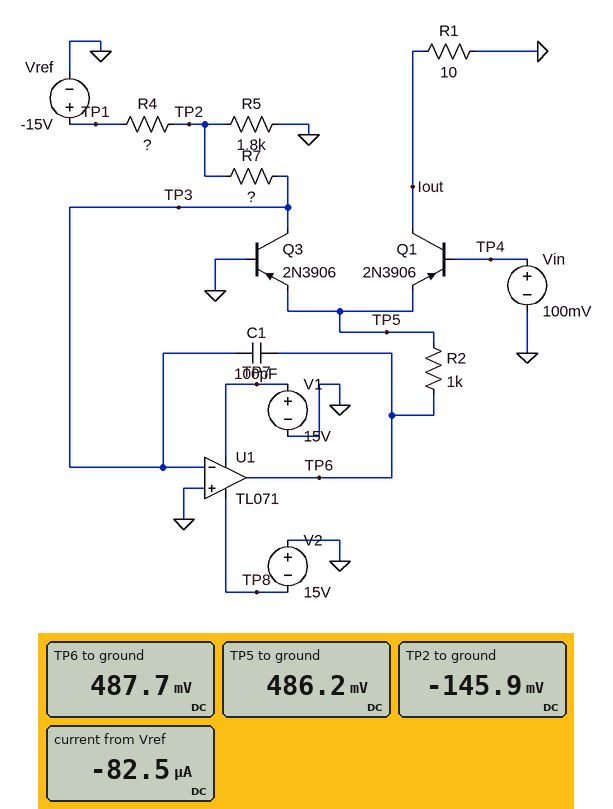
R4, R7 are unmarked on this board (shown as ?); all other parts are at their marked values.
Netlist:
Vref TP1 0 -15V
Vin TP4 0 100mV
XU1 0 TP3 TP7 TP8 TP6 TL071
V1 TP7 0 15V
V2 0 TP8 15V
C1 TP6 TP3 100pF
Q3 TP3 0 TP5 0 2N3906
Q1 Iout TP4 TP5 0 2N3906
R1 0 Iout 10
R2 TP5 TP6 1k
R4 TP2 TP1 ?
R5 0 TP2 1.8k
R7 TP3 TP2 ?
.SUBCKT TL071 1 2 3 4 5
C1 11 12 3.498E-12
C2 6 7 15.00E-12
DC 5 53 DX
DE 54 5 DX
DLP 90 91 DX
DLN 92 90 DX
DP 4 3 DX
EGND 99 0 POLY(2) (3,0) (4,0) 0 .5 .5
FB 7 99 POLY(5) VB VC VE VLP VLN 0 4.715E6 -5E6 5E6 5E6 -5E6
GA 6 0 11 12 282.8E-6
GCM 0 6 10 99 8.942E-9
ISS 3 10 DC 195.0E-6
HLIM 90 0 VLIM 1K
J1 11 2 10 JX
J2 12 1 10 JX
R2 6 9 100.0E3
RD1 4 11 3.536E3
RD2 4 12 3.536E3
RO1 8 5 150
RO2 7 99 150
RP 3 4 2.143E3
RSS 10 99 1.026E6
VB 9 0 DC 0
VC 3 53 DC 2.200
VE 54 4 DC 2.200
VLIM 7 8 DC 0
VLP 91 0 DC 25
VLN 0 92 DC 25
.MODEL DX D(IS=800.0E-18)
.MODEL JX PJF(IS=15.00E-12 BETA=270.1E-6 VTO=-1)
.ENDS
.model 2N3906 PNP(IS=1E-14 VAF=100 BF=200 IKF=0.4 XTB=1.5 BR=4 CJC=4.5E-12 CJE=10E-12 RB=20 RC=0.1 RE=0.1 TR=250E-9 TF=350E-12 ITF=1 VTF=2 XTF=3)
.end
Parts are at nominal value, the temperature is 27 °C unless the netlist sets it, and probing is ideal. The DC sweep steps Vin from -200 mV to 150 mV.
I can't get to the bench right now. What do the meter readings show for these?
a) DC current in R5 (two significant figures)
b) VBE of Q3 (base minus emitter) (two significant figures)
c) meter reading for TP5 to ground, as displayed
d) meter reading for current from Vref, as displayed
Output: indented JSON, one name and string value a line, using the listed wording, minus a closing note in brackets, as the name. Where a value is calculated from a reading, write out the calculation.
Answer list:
{
  "DC current in R5": "(0 V - (-145.9 mV)) / 1.8 kΩ = 81 µA",
  "VBE of Q3 (base minus emitter)": "0 V - 486.2 mV = -490 mV",
  "meter reading for TP5 to ground, as displayed": "486.2 mV",
  "meter reading for current from Vref, as displayed": "-82.5 µA"
}
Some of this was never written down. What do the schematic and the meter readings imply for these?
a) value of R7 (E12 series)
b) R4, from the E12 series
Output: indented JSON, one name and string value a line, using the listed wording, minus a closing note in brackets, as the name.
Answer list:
{
  "value of R7": "100 kΩ",
  "R4, from the E12 series": "180 kΩ"
}
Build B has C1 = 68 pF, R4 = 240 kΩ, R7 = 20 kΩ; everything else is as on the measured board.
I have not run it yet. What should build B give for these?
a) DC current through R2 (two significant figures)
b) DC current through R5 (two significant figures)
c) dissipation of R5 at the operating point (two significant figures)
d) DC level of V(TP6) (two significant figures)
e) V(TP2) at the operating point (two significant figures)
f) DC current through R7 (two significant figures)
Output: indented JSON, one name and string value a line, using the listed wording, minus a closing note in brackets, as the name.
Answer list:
{
  "DC current through R2": "5.3 µA",
  "DC current through R5": "57 µA",
  "dissipation of R5 at the operating point": "5.8 µW",
  "DC level of V(TP6)": "520 mV",
  "V(TP2) at the operating point": "-100 mV",
  "DC current through R7": "5.1 µA"
}
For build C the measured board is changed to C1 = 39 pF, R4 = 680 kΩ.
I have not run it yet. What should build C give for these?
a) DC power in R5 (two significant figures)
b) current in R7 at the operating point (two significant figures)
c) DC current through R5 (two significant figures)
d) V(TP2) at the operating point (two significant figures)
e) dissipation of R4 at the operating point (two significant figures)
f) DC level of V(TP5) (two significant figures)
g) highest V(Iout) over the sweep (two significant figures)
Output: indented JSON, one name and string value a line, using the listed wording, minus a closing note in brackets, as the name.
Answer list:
{
  "DC power in R5": "840 nW",
  "current in R7 at the operating point": "390 nA",
  "DC current through R5": "22 µA",
  "V(TP2) at the operating point": "-39 mV",
  "dissipation of R4 at the operating point": "330 µW",
  "DC level of V(TP5)": "450 mV",
  "highest V(Iout) over the sweep": "8.8 mV"
}
